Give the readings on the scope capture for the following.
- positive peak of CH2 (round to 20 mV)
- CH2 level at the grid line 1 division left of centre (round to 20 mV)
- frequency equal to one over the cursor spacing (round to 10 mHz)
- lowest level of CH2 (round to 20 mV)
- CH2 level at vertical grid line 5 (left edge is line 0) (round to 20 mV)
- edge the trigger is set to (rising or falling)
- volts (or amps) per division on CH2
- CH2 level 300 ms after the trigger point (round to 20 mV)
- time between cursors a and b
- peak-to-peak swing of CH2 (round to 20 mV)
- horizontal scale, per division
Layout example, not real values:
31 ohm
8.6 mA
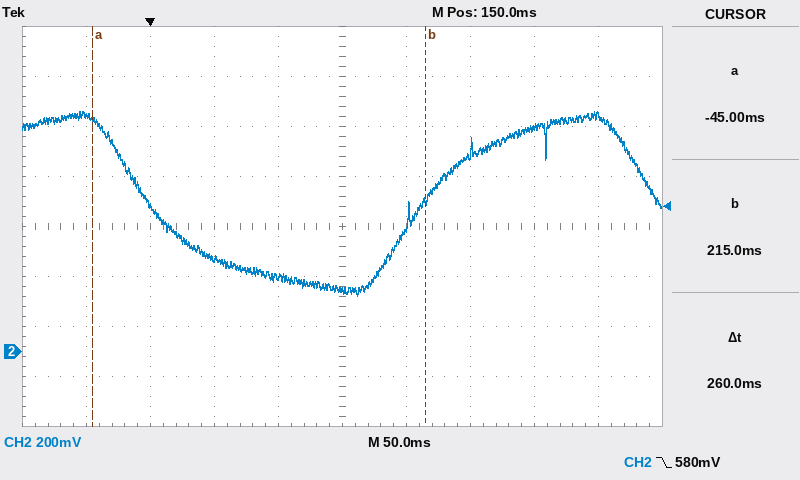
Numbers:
960 mV
300 mV
3.85 Hz
220 mV
240 mV
falling
200 mV
900 mV
260 ms
740 mV
50 ms
